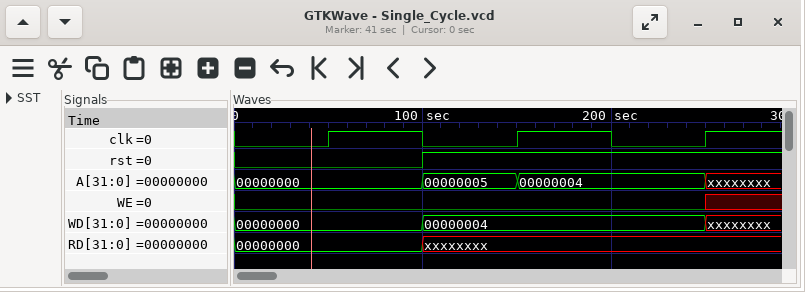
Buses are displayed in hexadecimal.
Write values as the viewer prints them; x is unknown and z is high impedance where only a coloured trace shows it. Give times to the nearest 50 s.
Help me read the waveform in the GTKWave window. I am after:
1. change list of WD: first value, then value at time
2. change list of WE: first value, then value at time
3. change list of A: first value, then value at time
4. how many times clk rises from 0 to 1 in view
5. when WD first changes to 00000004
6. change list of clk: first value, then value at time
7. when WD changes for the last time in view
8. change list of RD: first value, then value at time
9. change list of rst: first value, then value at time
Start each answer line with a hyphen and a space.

- 00000000, 00000004 at 100 s, xxxxxxxx at 250 s
- 0, x at 250 s
- 00000000, 00000005 at 100 s, 00000004 at 150 s, xxxxxxxx at 250 s
- 3
- 100 s
- 0, 1 at 50 s, 0 at 100 s, 1 at 150 s, 0 at 200 s, 1 at 250 s
- 250 s
- 00000000, xxxxxxxx at 100 s
- 0, 1 at 100 s
